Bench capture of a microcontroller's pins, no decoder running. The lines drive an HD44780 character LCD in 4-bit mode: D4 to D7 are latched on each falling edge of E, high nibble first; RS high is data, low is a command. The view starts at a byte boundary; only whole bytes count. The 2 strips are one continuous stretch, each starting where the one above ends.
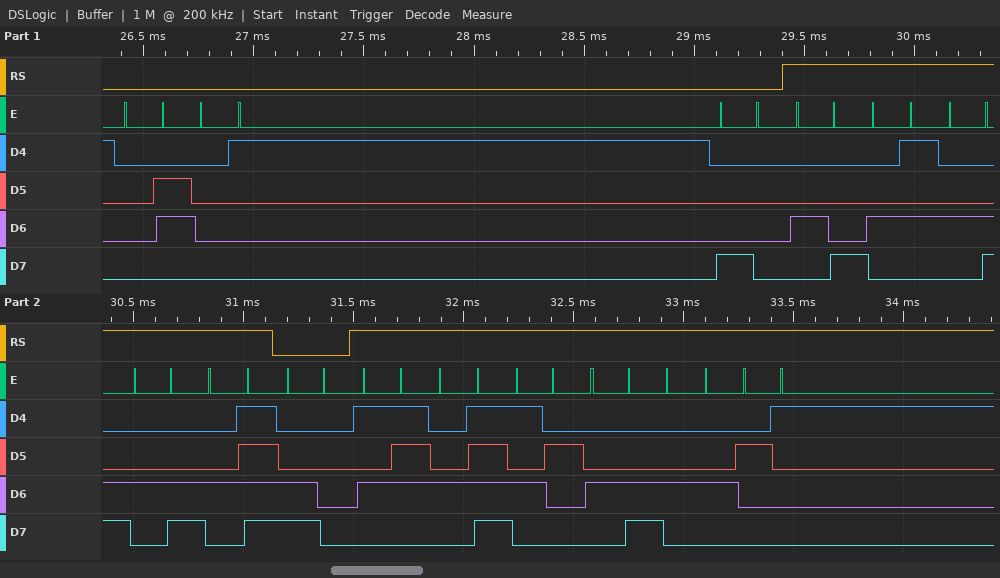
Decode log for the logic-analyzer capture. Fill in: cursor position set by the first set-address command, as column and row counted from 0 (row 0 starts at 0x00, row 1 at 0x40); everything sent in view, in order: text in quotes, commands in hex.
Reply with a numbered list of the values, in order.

1. column 0, row 0
2. 0x06 0x01 0x80 "HELLO" 0xC0 "WORLD!"
